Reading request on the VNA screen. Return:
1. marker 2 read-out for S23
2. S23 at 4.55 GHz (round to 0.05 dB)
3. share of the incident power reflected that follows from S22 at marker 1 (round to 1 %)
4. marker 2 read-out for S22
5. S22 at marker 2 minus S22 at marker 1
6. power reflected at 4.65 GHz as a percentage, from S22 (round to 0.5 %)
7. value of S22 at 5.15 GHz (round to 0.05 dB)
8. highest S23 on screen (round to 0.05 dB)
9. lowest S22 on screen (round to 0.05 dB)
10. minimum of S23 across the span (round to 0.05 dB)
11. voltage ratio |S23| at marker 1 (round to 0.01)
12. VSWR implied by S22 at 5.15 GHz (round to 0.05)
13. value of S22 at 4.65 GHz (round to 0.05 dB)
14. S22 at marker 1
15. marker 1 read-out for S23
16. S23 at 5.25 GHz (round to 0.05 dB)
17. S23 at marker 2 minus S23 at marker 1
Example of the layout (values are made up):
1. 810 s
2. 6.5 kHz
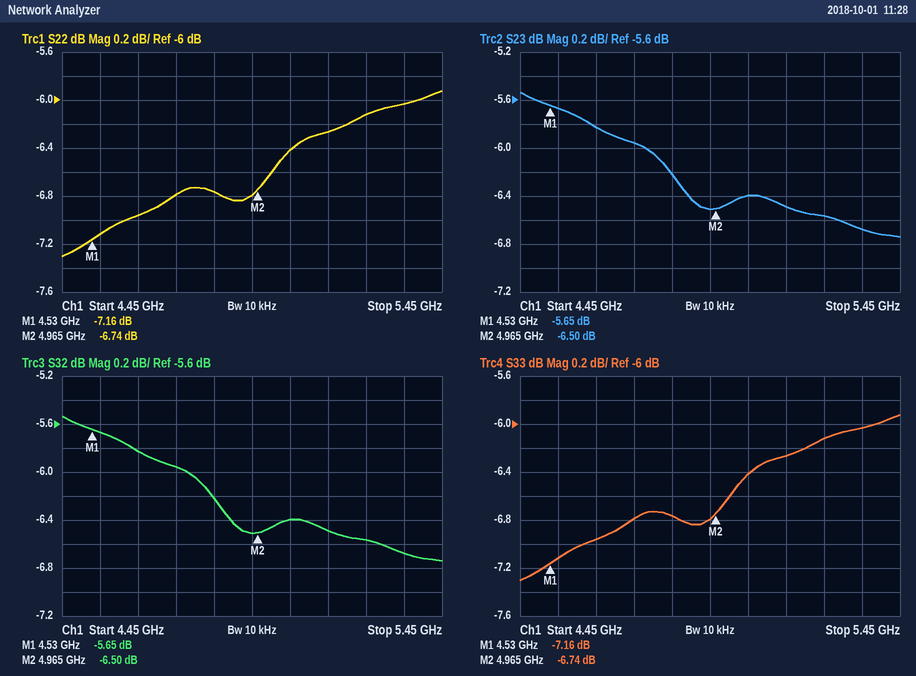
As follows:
1. -6.50 dB
2. -5.65 dB
3. 19 %
4. -6.74 dB
5. 0.42 dB
6. 20.0 %
7. -6.25 dB
8. -5.55 dB
9. -7.30 dB
10. -6.75 dB
11. 0.52
12. 2.90
13. -6.95 dB
14. -7.16 dB
15. -5.65 dB
16. -6.55 dB
17. -0.85 dB
